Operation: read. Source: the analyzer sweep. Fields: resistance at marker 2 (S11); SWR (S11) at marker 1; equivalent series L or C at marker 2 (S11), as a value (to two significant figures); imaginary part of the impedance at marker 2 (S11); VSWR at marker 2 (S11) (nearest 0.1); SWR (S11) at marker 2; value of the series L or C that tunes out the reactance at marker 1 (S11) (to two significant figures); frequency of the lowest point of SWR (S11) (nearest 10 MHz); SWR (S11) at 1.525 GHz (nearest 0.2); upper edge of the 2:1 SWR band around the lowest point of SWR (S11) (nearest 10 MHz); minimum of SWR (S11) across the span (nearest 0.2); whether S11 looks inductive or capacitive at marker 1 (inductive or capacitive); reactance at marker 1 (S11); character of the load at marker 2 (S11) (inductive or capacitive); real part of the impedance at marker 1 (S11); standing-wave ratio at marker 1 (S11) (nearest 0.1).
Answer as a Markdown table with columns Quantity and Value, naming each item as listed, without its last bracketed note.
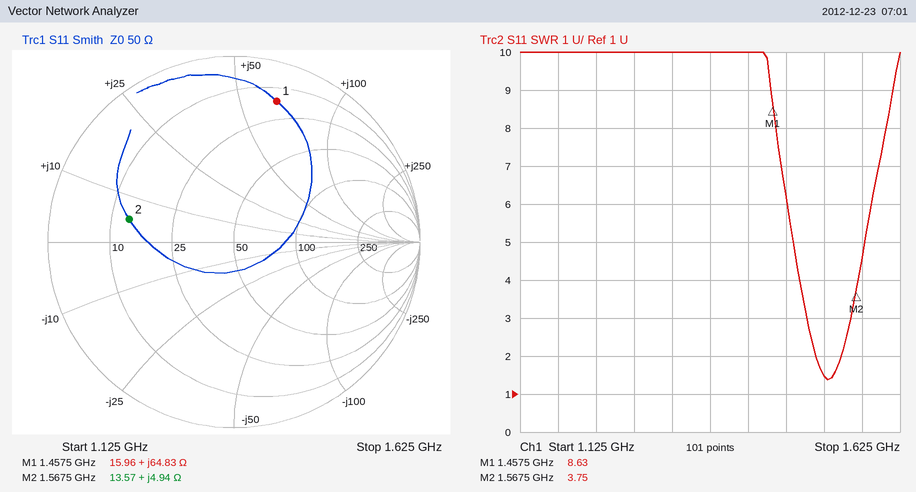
| Quantity | Value |
|---|---|
| resistance at marker 2 | 13.57 Ω |
| SWR (S11) at marker 1 | 8.63 |
| equivalent series L or C at marker 2 (S11), as a value | 500 pH |
| imaginary part of the impedance at marker 2 | +4.94 Ω |
| VSWR at marker 2 (S11) | 3.7 |
| SWR (S11) at marker 2 | 3.75 |
| value of the series L or C that tunes out the reactance at marker 1 (S11) | 1.7 pF |
| frequency of the lowest point of SWR (S11) | 1.53 GHz |
| SWR (S11) at 1.525 GHz | 1.4 |
| upper edge of the 2:1 SWR band around the lowest point of SWR (S11) | 1.55 GHz |
| minimum of SWR (S11) across the span | 1.4 |
| whether S11 looks inductive or capacitive at marker 1 | inductive |
| reactance at marker 1 | +64.83 Ω |
| character of the load at marker 2 (S11) | inductive |
| real part of the impedance at marker 1 | 15.96 Ω |
| standing-wave ratio at marker 1 (S11) | 8.6 |
